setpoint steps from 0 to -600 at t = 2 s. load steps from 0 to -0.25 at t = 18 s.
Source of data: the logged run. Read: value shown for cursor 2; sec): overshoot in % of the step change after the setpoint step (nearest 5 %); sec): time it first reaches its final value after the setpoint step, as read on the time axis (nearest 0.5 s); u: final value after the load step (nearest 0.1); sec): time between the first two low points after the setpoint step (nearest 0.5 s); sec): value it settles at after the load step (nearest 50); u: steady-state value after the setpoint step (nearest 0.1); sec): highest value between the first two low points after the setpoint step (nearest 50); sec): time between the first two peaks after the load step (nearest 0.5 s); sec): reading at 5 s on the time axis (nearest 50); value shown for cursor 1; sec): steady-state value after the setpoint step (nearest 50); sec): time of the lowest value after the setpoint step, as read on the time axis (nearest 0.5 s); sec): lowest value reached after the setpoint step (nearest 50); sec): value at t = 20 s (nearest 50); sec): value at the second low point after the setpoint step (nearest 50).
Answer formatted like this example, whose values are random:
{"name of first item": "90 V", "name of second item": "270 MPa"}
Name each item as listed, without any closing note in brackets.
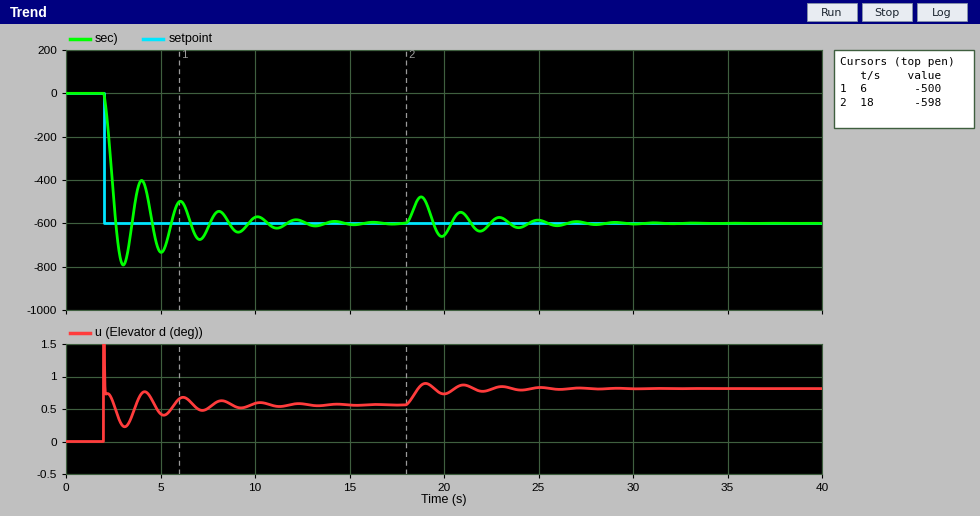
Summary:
{"value shown for cursor 2": "-598", "sec): overshoot in % of the step change after the setpoint step": "30 %", "sec): time it first reaches its final value after the setpoint step, as read on the time axis": "2.5 s", "u: final value after the load step": "0.8", "sec): time between the first two low points after the setpoint step": "2.0 s", "sec): value it settles at after the load step": "-600", "u: steady-state value after the setpoint step": "0.6", "sec): highest value between the first two low points after the setpoint step": "-400", "sec): time between the first two peaks after the load step": "2.0 s", "sec): reading at 5 s on the time axis": "-750", "value shown for cursor 1": "-500", "sec): steady-state value after the setpoint step": "-600", "sec): time of the lowest value after the setpoint step, as read on the time axis": "3.0 s", "sec): lowest value reached after the setpoint step": "-800", "sec): value at t = 20 s": "-650", "sec): value at the second low point after the setpoint step": "-750"}
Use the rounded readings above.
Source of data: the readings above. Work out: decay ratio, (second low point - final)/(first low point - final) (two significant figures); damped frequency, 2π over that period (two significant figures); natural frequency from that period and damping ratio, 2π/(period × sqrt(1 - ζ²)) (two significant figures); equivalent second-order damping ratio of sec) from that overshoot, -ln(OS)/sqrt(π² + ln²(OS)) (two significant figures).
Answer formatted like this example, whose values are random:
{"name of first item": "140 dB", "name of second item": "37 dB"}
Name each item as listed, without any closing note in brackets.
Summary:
{"decay ratio, (second low point - final)/(first low point - final)": "0.75", "damped frequency, 2π over that period": "3.1 rad/s", "natural frequency from that period and damping ratio, 2π/(period × sqrt(1 - ζ²))": "3.4 rad/s", "equivalent second-order damping ratio of sec) from that overshoot, -ln(OS)/sqrt(π² + ln²(OS))": "0.36"}
